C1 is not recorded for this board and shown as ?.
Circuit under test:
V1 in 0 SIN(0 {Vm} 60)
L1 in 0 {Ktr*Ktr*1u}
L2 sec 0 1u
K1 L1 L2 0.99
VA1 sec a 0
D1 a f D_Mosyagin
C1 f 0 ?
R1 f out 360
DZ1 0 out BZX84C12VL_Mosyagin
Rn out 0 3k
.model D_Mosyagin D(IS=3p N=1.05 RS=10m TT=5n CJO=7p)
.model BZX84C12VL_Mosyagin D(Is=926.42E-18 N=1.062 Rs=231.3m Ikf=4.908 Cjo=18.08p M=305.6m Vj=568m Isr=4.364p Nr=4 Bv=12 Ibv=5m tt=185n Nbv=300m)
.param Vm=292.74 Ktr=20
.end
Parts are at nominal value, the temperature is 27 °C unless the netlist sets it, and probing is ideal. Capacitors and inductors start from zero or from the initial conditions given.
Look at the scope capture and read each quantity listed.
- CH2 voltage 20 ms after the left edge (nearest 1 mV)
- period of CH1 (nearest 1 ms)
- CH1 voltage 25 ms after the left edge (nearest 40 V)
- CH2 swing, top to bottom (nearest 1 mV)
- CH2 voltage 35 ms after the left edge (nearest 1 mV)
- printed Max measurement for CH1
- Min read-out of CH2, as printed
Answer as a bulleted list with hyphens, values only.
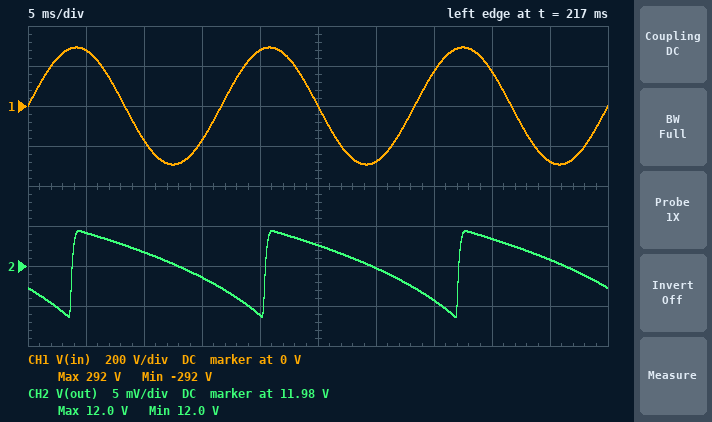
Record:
- 11.979 V
- 17 ms
- 0 V
- 11 mV
- 11.981 V
- 292 V
- 12.0 V
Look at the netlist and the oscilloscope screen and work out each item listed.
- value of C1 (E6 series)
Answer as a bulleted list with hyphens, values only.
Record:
- 220 µF
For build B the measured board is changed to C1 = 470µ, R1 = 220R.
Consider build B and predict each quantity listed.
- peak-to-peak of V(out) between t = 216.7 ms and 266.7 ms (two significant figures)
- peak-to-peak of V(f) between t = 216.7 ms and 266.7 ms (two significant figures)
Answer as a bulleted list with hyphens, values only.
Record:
- 2.7 mV
- 260 mV
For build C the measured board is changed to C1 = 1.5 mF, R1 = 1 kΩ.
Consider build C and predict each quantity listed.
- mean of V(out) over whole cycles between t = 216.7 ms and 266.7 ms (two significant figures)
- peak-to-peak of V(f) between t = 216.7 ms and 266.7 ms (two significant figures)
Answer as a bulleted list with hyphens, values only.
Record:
- 10 V
- 37 mV
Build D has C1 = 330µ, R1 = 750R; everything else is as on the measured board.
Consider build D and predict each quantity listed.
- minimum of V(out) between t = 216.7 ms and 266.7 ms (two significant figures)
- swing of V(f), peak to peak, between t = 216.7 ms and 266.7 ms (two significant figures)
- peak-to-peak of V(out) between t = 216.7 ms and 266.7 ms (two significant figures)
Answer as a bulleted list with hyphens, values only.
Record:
- 11 V
- 180 mV
- 140 mV
